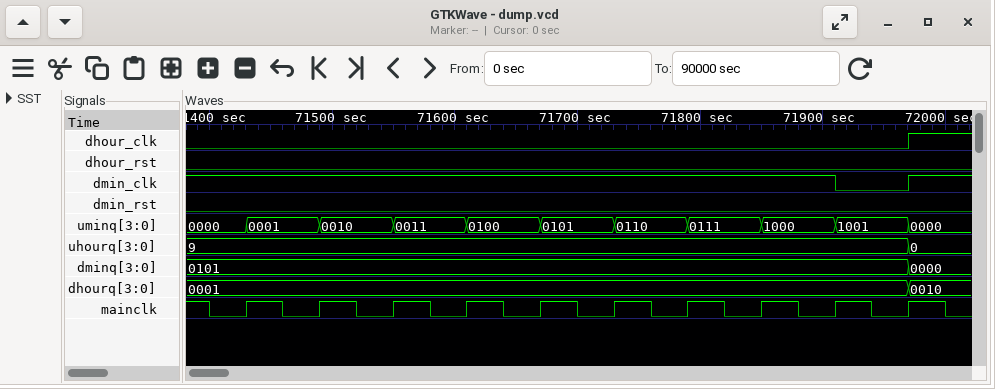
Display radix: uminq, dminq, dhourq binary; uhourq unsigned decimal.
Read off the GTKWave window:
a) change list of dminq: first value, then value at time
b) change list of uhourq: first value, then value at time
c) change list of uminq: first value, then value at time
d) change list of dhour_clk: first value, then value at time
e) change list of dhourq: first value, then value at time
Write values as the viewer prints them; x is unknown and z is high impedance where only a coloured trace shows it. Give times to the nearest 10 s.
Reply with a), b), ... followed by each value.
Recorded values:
a) 0101, 0000 at 71970 s
b) 9, 0 at 71970 s
c) 0000, 0001 at 71430 s, 0010 at 71490 s, 0011 at 71550 s, 0100 at 71610 s, 0101 at 71670 s, 0110 at 71730 s, 0111 at 71790 s, 1000 at 71850 s, 1001 at 71910 s, 0000 at 71970 s
d) 0, 1 at 71970 s
e) 0001, 0010 at 71970 s
